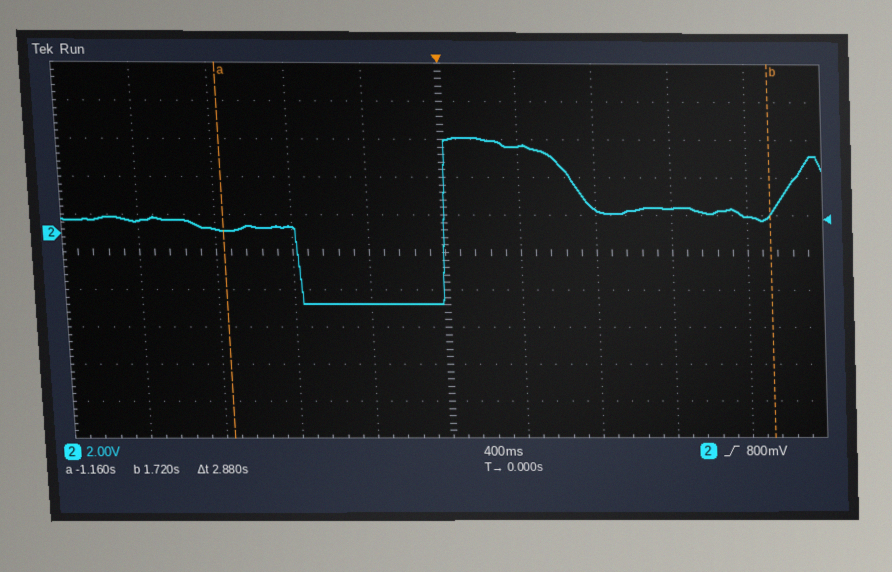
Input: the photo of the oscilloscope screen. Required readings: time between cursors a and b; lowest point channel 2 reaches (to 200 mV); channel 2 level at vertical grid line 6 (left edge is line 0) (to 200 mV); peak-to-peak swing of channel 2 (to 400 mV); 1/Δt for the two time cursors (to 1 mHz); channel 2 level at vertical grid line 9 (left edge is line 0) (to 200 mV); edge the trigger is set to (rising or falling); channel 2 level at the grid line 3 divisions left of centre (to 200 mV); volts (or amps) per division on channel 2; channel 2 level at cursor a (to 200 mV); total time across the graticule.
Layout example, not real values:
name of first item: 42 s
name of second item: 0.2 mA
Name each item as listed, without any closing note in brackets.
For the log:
time between cursors a and b: 2.88 s
lowest point channel 2 reaches: -3.8 V
channel 2 level at vertical grid line 6 (left edge is line 0): 4.6 V
peak-to-peak swing of channel 2: 8.8 V
1/Δt for the two time cursors: 347 mHz
channel 2 level at vertical grid line 9 (left edge is line 0): 1.0 V
edge the trigger is set to: rising
channel 2 level at the grid line 3 divisions left of centre: 200 mV
volts (or amps) per division on channel 2: 2 V
channel 2 level at cursor a: 200 mV
total time across the graticule: 4 s
